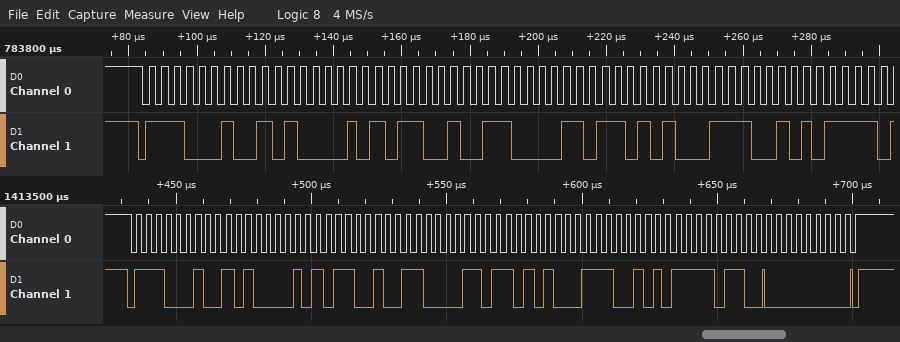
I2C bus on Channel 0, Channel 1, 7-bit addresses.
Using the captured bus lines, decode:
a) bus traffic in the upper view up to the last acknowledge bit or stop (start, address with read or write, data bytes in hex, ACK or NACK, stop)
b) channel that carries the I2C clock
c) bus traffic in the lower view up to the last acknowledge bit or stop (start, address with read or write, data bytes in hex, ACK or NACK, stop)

start, address 71 write ACK, A1 ACK, B2 ACK, C3 ACK, D4 ACK, E5 ACK
Channel 0
start, address 71 write ACK, A1 ACK, B2 ACK, C3 ACK, D4 ACK, E5 ACK, F6 ACK, 00 ACK, stop
